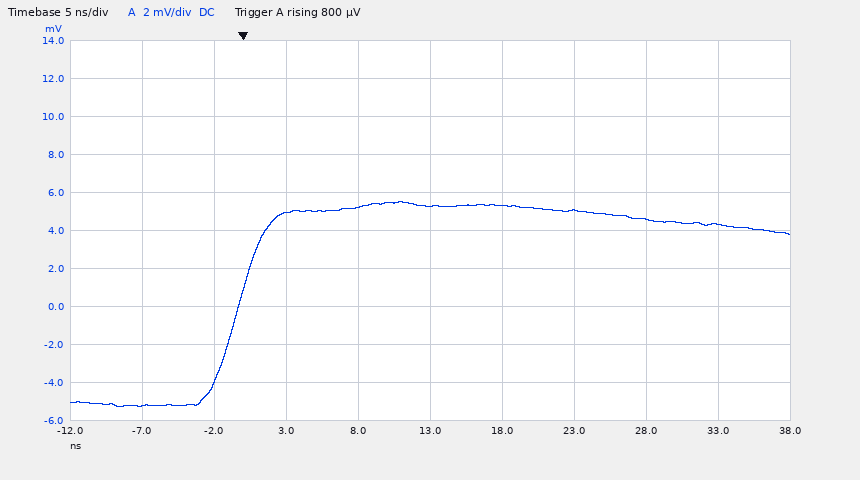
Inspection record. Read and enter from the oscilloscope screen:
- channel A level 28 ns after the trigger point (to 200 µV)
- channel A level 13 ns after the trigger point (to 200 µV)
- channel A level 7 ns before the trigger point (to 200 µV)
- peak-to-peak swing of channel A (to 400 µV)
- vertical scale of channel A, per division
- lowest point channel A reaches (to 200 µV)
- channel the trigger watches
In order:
4.6 mV
5.2 mV
-5.2 mV
10.8 mV
2 mV
-5.2 mV
channel A
